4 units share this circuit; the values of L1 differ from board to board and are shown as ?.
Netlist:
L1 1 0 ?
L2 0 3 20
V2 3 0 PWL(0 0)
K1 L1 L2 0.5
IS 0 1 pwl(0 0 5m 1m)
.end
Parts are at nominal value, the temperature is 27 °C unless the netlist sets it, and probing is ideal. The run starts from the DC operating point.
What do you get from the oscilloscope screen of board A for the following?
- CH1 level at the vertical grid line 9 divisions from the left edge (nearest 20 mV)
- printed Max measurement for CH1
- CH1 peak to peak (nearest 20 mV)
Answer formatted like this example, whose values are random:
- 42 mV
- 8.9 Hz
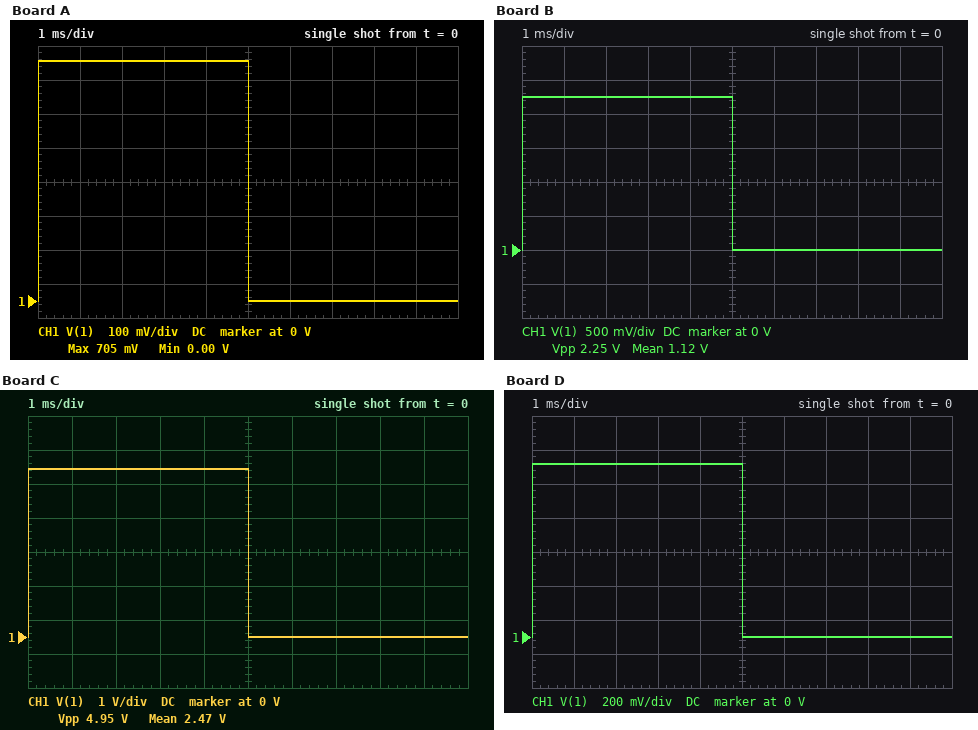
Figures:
- 0 V
- 705 mV
- 700 mV
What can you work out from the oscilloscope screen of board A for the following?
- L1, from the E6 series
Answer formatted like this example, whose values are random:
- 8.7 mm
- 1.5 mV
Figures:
- 4.7 H
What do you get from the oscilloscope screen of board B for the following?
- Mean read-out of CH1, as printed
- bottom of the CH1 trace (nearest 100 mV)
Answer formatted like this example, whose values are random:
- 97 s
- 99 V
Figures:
- 1.12 V
- 0 V
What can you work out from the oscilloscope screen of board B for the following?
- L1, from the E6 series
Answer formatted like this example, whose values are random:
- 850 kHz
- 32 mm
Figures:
- 15 H
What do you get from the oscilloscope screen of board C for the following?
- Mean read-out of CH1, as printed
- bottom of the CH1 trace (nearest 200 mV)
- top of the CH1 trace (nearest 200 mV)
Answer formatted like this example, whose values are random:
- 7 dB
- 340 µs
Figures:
- 2.47 V
- 0 V
- 5.0 V
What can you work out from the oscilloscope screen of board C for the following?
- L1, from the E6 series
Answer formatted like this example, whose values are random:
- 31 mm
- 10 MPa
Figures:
- 33 H
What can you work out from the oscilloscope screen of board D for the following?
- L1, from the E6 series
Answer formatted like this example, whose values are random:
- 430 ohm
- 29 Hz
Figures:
- 6.8 H
